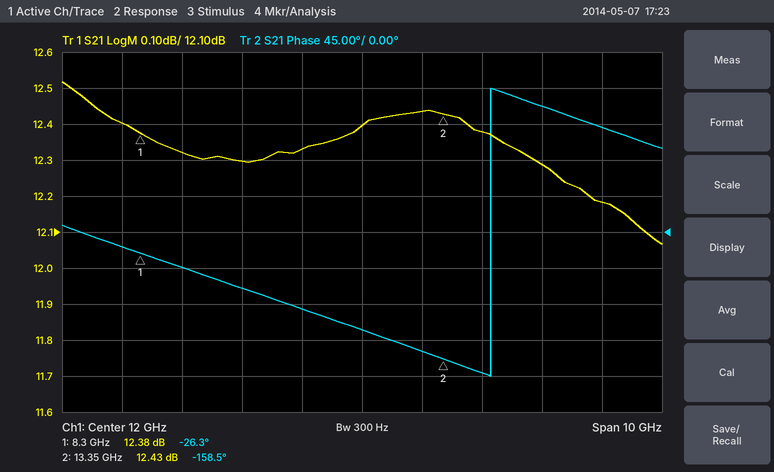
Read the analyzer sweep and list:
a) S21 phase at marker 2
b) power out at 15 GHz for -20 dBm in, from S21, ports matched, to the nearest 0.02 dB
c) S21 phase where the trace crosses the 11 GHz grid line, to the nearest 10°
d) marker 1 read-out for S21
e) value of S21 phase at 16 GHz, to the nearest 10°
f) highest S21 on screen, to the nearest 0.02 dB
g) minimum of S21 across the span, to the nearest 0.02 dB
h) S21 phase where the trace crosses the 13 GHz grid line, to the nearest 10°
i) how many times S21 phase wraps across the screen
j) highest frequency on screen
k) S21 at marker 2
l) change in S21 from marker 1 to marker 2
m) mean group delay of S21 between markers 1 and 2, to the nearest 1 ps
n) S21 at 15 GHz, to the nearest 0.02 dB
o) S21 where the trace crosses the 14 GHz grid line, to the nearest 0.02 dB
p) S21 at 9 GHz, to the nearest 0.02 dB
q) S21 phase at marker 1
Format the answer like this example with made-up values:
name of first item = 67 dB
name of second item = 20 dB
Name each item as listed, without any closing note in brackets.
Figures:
S21 phase at marker 2 = -158.5°
power out at 15 GHz for -20 dBm in, from S21, ports matched, to the nearest 0.02 dB = -7.72 dBm
S21 phase where the trace crosses the 11 GHz grid line, to the nearest 10° = -100°
marker 1 read-out for S21 = 12.38 dB
value of S21 phase at 16 GHz, to the nearest 10° = 130°
highest S21 on screen, to the nearest 0.02 dB = 12.52 dB
minimum of S21 across the span, to the nearest 0.02 dB = 12.06 dB
S21 phase where the trace crosses the 13 GHz grid line, to the nearest 10° = -150°
how many times S21 phase wraps across the screen = 1
highest frequency on screen = 17 GHz
S21 at marker 2 = 12.43 dB
change in S21 from marker 1 to marker 2 = 0.05 dB
mean group delay of S21 between markers 1 and 2, to the nearest 1 ps = 73 ps
S21 at 15 GHz, to the nearest 0.02 dB = 12.28 dB
S21 where the trace crosses the 14 GHz grid line, to the nearest 0.02 dB = 12.38 dB
S21 at 9 GHz, to the nearest 0.02 dB = 12.32 dB
S21 phase at marker 1 = -26.3°
